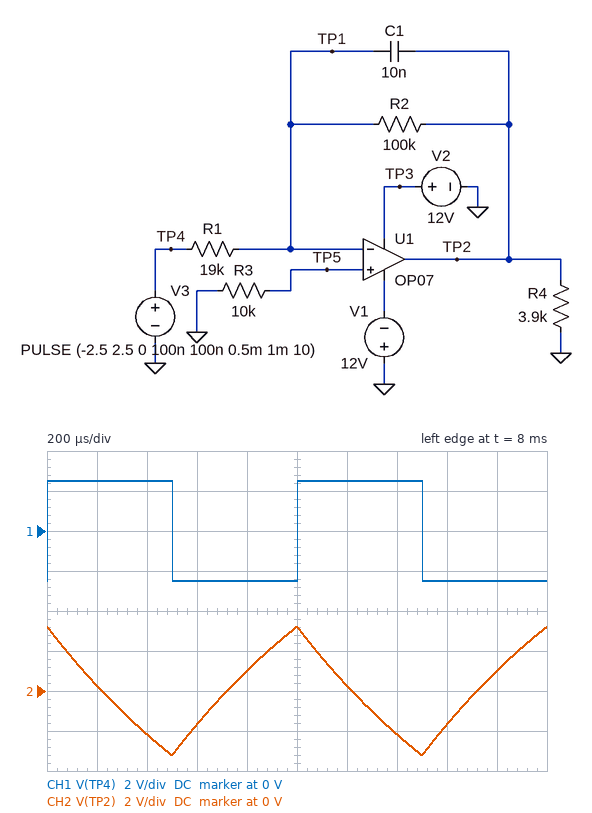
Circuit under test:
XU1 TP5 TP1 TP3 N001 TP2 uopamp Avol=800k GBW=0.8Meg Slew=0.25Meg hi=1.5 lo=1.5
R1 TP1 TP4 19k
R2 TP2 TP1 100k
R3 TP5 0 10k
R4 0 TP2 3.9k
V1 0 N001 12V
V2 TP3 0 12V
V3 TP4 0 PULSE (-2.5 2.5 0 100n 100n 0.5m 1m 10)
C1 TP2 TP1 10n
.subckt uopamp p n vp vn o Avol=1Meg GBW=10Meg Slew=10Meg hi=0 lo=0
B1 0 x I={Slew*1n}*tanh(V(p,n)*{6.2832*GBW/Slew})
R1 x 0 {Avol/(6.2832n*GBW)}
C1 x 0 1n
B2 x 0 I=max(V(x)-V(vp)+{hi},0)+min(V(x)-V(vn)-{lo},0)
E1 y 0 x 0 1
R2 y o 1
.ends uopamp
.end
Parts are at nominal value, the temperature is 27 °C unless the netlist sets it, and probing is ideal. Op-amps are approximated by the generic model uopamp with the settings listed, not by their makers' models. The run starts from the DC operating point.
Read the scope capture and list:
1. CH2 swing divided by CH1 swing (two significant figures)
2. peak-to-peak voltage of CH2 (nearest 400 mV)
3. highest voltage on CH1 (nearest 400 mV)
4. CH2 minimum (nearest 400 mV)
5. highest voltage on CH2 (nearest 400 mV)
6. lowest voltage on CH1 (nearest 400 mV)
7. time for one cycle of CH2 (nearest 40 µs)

1.3
6.4 V
2.4 V
-3.2 V
3.2 V
-2.4 V
1.00 ms
